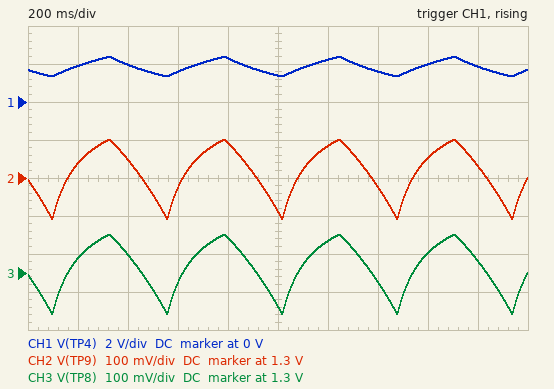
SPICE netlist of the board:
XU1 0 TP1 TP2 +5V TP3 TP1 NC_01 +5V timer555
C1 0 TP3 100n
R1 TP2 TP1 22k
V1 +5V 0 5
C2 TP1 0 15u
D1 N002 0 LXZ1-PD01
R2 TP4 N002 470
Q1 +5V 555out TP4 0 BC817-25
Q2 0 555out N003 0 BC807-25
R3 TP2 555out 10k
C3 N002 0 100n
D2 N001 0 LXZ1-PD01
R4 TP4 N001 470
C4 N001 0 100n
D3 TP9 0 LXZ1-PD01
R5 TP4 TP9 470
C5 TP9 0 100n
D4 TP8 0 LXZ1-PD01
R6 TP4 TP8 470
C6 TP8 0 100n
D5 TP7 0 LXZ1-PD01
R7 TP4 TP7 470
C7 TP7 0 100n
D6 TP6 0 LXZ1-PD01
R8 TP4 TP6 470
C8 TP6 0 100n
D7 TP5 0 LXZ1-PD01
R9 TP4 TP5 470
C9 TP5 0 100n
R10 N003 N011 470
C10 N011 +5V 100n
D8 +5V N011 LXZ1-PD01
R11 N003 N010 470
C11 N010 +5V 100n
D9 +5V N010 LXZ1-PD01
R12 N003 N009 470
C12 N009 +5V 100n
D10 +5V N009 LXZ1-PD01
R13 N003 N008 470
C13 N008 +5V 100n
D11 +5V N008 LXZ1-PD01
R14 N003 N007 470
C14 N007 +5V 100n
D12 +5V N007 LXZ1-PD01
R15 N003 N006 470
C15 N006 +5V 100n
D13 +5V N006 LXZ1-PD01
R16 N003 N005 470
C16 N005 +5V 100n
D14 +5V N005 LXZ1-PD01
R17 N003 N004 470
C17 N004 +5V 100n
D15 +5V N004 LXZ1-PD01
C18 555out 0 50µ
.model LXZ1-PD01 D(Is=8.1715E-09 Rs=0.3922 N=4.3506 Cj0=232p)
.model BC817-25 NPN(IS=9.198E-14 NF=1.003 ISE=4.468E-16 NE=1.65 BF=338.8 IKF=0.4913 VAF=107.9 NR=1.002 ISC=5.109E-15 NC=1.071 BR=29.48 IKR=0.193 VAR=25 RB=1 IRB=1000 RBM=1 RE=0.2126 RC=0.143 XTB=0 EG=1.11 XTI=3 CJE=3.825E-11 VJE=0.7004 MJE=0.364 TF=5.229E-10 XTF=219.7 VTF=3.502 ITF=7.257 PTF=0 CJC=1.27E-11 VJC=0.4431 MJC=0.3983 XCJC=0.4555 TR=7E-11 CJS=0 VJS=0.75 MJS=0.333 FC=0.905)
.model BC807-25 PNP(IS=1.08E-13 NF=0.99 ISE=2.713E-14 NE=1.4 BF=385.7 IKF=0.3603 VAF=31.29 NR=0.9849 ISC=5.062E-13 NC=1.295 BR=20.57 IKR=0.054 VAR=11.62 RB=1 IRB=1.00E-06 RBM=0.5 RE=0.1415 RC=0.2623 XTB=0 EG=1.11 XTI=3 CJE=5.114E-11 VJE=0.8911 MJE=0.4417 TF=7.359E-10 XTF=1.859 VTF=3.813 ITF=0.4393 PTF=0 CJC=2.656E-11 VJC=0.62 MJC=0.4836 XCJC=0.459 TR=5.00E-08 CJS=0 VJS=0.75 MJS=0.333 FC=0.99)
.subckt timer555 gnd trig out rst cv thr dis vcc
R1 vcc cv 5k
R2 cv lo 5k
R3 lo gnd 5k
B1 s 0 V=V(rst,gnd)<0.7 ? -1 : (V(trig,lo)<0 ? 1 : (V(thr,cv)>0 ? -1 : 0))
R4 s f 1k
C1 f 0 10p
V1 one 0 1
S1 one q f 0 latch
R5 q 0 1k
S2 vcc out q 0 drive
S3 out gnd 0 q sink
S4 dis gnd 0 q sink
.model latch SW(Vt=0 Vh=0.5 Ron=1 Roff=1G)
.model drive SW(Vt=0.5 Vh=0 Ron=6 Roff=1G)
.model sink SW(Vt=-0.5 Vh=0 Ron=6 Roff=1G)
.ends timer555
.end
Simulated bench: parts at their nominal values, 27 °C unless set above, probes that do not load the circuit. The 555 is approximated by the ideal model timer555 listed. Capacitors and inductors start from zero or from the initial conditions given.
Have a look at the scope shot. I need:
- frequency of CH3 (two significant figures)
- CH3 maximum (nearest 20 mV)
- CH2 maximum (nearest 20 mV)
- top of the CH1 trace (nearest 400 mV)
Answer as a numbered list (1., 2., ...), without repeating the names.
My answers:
1. 2.2 Hz
2. 1.40 V
3. 1.40 V
4. 2.4 V
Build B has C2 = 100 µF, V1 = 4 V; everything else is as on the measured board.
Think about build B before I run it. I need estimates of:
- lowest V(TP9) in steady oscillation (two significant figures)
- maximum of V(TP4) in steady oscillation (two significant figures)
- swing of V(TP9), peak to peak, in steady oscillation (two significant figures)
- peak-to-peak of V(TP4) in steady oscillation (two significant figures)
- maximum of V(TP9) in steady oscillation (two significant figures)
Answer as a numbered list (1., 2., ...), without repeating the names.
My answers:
1. 270 mV
2. 2.7 V
3. 1.2 V
4. 2.4 V
5. 1.4 V
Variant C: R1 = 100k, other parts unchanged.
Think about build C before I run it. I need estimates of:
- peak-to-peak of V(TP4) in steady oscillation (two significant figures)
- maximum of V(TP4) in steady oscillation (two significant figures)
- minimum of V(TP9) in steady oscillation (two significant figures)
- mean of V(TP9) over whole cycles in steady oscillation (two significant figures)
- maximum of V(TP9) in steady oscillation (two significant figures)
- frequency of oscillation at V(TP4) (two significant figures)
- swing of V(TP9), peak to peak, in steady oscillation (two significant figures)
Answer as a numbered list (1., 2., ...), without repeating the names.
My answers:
1. 2.7 V
2. 3.3 V
3. 600 mV
4. 1.2 V
5. 1.5 V
6. 480 mHz
7. 870 mV
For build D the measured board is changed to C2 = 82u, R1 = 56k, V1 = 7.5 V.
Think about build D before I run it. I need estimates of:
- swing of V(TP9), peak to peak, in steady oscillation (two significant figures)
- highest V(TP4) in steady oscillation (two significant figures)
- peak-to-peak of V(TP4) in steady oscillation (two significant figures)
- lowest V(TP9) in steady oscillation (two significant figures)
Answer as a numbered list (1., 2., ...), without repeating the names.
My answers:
1. 430 mV
2. 5.1 V
3. 3.9 V
4. 1.1 V
